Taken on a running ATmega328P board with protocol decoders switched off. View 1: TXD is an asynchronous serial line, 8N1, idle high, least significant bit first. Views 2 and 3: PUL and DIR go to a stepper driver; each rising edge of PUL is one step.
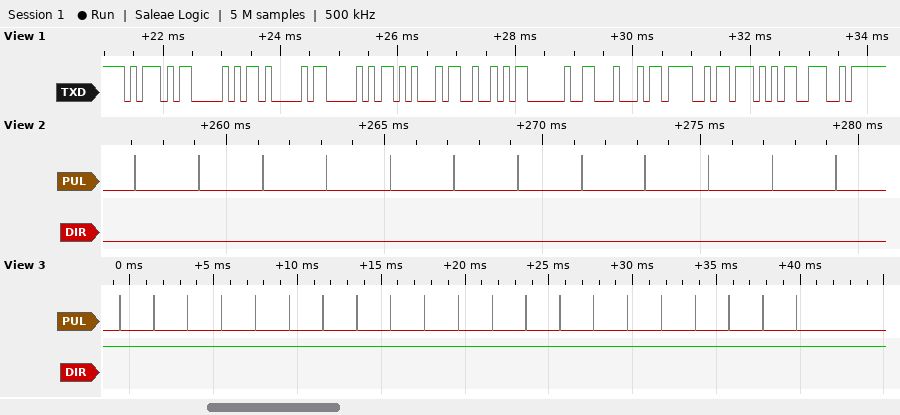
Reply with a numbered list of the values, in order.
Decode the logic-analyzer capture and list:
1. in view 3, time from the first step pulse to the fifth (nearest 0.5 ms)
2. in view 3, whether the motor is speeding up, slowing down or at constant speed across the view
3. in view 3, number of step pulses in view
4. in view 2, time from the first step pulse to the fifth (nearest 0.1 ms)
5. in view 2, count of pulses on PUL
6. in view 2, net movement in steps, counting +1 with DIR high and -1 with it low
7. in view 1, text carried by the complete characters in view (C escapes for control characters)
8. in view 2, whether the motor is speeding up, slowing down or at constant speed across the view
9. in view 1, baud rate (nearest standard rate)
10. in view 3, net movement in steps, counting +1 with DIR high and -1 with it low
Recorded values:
1. 8.0 ms
2. constant speed
3. 21
4. 8.1 ms
5. 12
6. -12
7. "]PAPER DOWN"
8. constant speed
9. 9600 baud
10. +21
